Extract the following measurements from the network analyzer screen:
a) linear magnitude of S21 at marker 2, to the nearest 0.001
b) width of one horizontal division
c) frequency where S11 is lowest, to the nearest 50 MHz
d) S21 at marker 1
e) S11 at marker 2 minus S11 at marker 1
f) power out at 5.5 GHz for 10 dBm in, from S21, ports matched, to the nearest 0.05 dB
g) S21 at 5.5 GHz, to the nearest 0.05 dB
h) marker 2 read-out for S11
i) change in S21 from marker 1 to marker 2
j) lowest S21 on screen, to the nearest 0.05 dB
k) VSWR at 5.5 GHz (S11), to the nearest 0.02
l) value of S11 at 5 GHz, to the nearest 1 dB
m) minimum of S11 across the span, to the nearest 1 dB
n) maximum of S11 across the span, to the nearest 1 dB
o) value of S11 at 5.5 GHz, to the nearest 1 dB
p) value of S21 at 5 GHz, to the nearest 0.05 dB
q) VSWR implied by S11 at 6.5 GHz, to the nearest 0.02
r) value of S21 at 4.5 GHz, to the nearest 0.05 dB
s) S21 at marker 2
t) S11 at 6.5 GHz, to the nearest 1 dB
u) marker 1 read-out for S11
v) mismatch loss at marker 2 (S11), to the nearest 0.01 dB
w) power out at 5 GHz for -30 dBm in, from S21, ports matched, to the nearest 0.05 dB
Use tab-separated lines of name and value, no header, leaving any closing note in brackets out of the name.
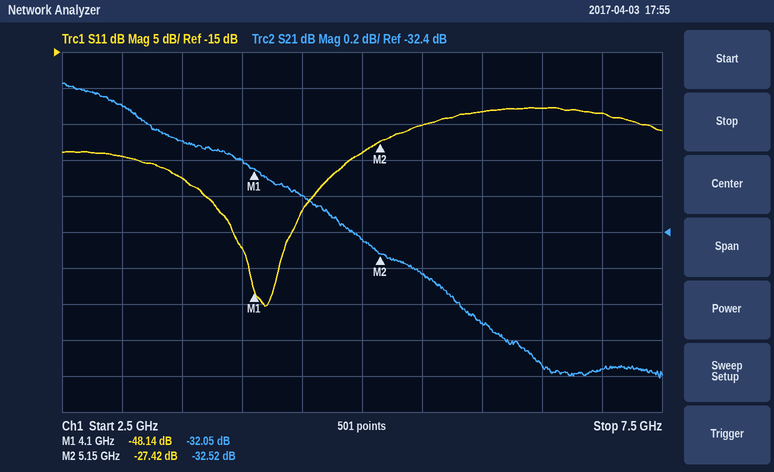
linear magnitude of S21 at marker 2, to the nearest 0.001	0.024
width of one horizontal division	500 MHz
frequency where S11 is lowest, to the nearest 50 MHz	4.20 GHz
S21 at marker 1	-32.05 dB
S11 at marker 2 minus S11 at marker 1	20.72 dB
power out at 5.5 GHz for 10 dBm in, from S21, ports matched, to the nearest 0.05 dB	-22.65 dBm
S21 at 5.5 GHz, to the nearest 0.05 dB	-32.65 dB
marker 2 read-out for S11	-27.42 dB
change in S21 from marker 1 to marker 2	-0.47 dB
lowest S21 on screen, to the nearest 0.05 dB	-33.20 dB
VSWR at 5.5 GHz (S11), to the nearest 0.02	1.12
value of S11 at 5 GHz, to the nearest 1 dB	-29 dB
minimum of S11 across the span, to the nearest 1 dB	-50 dB
maximum of S11 across the span, to the nearest 1 dB	-23 dB
value of S11 at 5.5 GHz, to the nearest 1 dB	-25 dB
value of S21 at 5 GHz, to the nearest 0.05 dB	-32.45 dB
VSWR implied by S11 at 6.5 GHz, to the nearest 0.02	1.16
value of S21 at 4.5 GHz, to the nearest 0.05 dB	-32.20 dB
S21 at marker 2	-32.52 dB
S11 at 6.5 GHz, to the nearest 1 dB	-23 dB
marker 1 read-out for S11	-48.14 dB
mismatch loss at marker 2 (S11), to the nearest 0.01 dB	0.01 dB
power out at 5 GHz for -30 dBm in, from S21, ports matched, to the nearest 0.05 dB	-62.45 dBm
